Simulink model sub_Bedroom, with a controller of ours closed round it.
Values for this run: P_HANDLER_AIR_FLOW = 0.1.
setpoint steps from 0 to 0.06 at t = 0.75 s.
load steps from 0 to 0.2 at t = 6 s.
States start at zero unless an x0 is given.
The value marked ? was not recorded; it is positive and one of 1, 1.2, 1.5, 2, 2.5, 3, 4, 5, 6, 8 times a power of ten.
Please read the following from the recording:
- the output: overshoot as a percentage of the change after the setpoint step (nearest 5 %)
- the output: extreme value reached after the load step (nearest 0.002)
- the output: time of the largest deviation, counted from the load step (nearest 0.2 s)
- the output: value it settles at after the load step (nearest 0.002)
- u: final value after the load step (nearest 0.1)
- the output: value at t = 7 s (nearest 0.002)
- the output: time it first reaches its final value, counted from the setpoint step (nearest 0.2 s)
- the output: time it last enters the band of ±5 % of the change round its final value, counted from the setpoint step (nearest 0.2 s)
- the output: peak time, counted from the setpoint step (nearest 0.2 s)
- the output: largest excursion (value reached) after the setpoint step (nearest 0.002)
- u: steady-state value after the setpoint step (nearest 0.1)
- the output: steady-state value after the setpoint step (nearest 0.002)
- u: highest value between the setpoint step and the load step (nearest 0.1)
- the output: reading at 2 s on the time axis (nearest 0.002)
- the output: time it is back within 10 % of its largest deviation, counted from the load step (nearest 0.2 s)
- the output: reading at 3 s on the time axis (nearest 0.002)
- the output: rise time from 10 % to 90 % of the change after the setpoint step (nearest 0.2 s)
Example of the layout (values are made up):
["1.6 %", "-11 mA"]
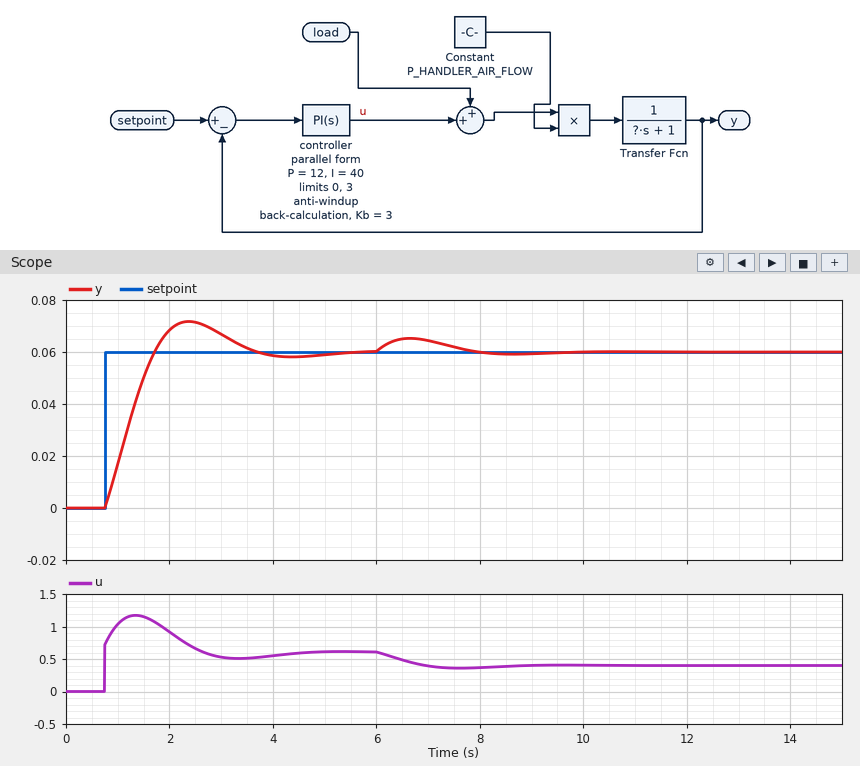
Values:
["20 %", "0.066", "0.6 s", "0.060", "0.4", "0.064", "1.0 s", "2.6 s", "1.6 s", "0.072", "0.6", "0.060", "1.2", "0.068", "3.2 s", "0.066", "0.8 s"]
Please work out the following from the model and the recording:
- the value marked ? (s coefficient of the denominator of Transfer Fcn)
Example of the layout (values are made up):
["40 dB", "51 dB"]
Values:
["1.2"]
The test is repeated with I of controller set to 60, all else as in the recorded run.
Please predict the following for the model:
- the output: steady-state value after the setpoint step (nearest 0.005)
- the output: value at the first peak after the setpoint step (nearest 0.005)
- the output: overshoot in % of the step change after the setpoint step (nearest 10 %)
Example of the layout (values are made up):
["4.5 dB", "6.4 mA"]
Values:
["0.060", "0.075", "30 %"]
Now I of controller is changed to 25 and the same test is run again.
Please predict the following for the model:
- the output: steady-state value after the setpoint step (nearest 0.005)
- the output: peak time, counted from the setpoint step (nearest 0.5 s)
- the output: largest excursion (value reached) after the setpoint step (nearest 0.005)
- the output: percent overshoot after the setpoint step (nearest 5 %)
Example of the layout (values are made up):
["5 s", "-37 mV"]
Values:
["0.060", "2.0 s", "0.065", "10 %"]
